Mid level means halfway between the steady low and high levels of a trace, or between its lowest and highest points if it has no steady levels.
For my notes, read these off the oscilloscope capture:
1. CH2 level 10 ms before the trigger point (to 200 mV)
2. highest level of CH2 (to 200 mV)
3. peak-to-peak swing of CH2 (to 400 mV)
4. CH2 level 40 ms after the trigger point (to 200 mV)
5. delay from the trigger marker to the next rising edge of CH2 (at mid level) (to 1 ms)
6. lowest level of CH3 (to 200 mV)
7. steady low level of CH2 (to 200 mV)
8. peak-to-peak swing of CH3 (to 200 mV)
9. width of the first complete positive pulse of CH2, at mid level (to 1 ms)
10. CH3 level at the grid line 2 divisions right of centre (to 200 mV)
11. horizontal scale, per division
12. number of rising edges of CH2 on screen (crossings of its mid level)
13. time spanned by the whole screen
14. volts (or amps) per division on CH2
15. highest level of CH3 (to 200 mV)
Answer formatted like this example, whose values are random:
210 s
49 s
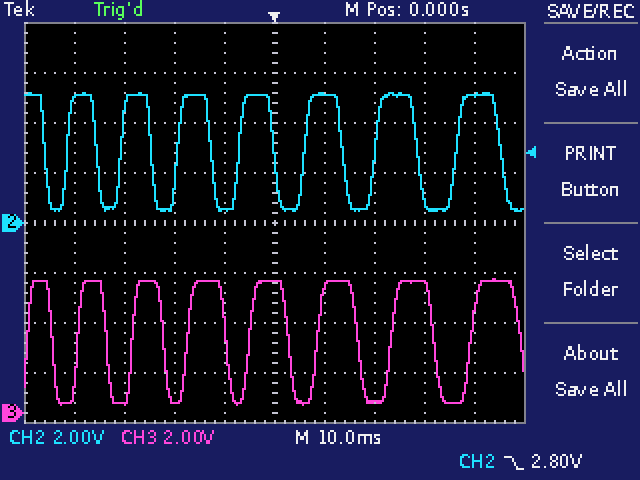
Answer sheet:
600 mV
5.2 V
4.8 V
5.2 V
6 ms
400 mV
600 mV
5.0 V
6 ms
400 mV
10 ms
7
100 ms
2 V
5.4 V
